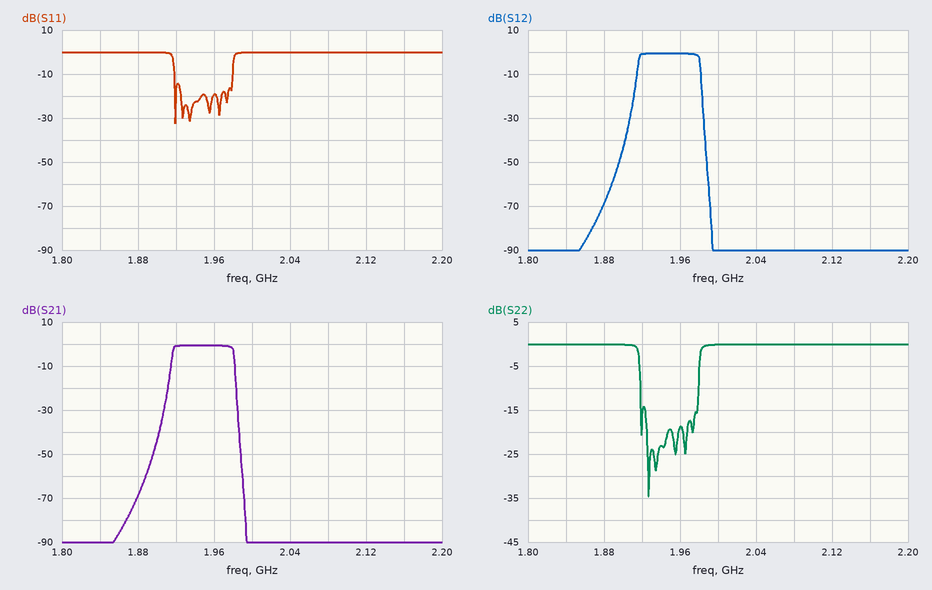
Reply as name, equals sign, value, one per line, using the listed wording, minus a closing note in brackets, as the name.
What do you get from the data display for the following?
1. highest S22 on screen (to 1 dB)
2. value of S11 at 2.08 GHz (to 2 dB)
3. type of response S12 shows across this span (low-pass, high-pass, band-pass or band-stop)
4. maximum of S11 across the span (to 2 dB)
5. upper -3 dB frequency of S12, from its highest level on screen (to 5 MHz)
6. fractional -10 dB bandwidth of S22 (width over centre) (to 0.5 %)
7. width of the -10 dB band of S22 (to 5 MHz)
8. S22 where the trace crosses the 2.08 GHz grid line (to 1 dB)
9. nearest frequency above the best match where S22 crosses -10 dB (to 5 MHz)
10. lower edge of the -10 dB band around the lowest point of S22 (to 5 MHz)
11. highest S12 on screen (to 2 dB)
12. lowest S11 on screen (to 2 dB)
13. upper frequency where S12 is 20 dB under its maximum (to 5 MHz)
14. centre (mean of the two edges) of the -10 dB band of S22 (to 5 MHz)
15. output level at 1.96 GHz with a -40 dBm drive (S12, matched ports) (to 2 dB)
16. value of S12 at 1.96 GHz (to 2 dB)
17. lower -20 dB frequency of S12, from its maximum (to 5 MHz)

highest S22 on screen = 0 dB
value of S11 at 2.08 GHz = 0 dB
type of response S12 shows across this span = band-pass
maximum of S11 across the span = 0 dB
upper -3 dB frequency of S12, from its highest level on screen = 1.980 GHz
fractional -10 dB bandwidth of S22 (width over centre) = 3.0 %
width of the -10 dB band of S22 = 60 MHz
S22 where the trace crosses the 2.08 GHz grid line = 0 dB
nearest frequency above the best match where S22 crosses -10 dB = 1.980 GHz
lower edge of the -10 dB band around the lowest point of S22 = 1.920 GHz
highest S12 on screen = 0 dB
lowest S11 on screen = -32 dB
upper frequency where S12 is 20 dB under its maximum = 1.985 GHz
centre (mean of the two edges) of the -10 dB band of S22 = 1.950 GHz
output level at 1.96 GHz with a -40 dBm drive (S12, matched ports) = -40 dBm
value of S12 at 1.96 GHz = 0 dB
lower -20 dB frequency of S12, from its maximum = 1.910 GHz
